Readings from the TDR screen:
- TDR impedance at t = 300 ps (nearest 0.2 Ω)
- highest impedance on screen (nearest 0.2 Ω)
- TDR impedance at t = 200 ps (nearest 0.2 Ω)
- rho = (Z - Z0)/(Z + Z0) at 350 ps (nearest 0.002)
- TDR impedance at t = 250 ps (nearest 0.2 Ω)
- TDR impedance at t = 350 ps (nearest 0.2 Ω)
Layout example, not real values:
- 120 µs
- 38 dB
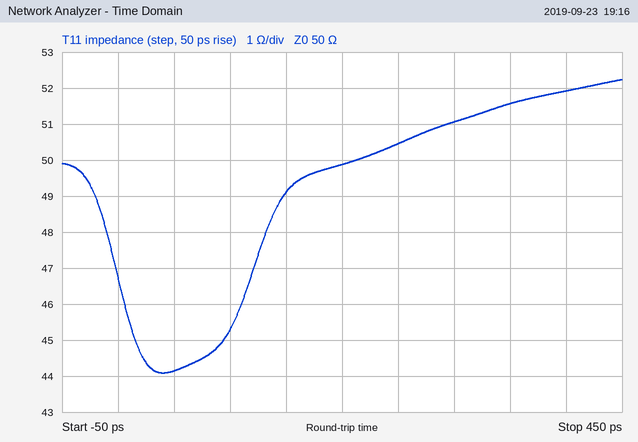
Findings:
- 51.0 Ω
- 52.2 Ω
- 49.8 Ω
- +0.016
- 50.4 Ω
- 51.6 Ω
